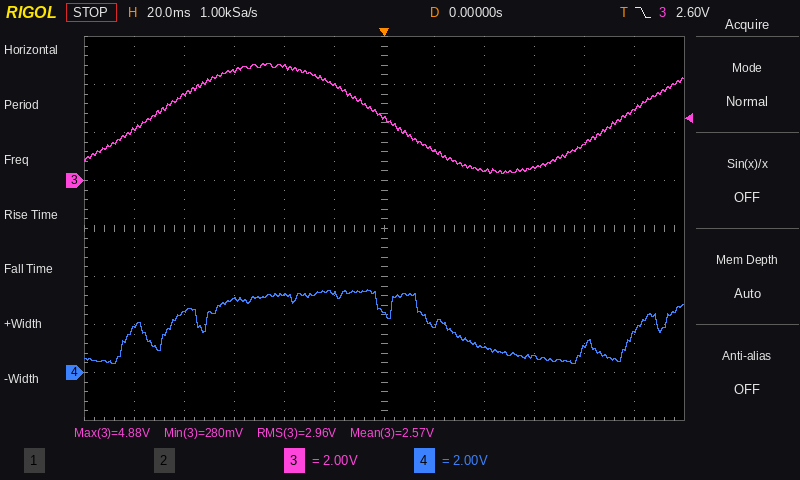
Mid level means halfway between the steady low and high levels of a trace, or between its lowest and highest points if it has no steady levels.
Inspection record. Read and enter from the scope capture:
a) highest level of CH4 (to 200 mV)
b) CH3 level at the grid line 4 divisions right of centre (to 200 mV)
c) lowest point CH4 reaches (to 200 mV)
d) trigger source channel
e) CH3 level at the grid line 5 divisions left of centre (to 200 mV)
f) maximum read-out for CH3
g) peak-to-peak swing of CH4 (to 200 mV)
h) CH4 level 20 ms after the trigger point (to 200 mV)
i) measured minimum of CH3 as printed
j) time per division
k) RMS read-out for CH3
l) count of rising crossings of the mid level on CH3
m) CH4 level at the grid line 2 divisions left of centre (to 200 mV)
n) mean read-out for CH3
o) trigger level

3.4 V
1.6 V
400 mV
CH3
2.2 V
4.88 V
3.0 V
2.0 V
280 mV
20 ms
2.96 V
2
3.2 V
2.57 V
2.60 V
